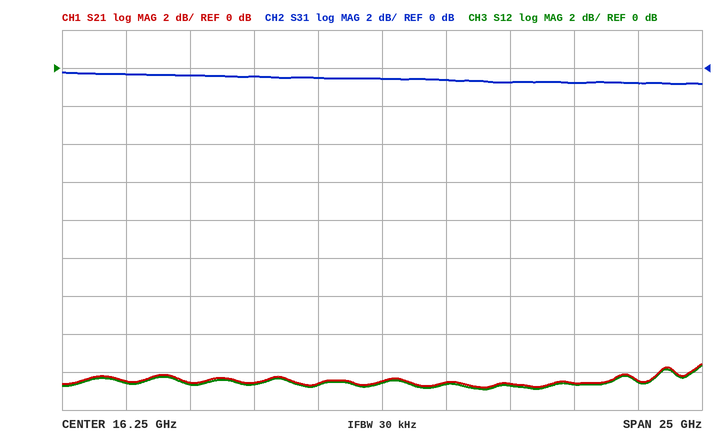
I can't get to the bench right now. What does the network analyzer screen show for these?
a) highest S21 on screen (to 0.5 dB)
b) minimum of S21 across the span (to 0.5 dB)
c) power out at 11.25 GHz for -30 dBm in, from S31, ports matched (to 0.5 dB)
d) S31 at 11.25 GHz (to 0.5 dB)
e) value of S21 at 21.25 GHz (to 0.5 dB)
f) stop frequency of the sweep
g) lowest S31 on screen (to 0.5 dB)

-15.5 dB
-17.0 dB
-30.5 dBm
-0.5 dB
-16.5 dB
28.75 GHz
-1.0 dB
